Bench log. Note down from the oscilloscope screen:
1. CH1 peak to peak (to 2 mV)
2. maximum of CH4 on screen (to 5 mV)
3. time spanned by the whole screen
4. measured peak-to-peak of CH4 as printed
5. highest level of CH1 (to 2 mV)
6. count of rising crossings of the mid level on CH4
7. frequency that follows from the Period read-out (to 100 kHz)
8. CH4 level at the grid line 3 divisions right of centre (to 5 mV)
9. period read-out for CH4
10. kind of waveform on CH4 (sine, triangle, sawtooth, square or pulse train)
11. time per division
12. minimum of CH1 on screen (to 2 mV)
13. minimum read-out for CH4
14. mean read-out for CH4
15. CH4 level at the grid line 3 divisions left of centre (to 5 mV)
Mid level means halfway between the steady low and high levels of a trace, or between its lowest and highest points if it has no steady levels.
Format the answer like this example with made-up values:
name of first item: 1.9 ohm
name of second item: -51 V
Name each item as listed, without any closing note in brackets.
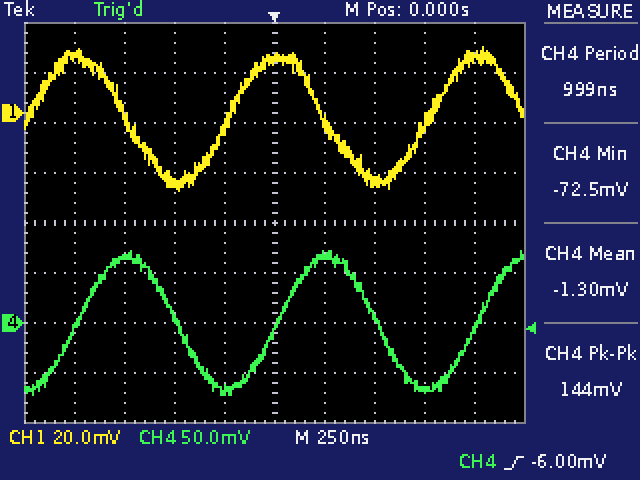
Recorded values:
CH1 peak to peak: 58 mV
maximum of CH4 on screen: 70 mV
time spanned by the whole screen: 2.5 µs
measured peak-to-peak of CH4 as printed: 144 mV
highest level of CH1: 26 mV
count of rising crossings of the mid level on CH4: 3
frequency that follows from the Period read-out: 1.0 MHz
CH4 level at the grid line 3 divisions right of centre: -65 mV
period read-out for CH4: 999 ns
kind of waveform on CH4: sine
time per division: 250 ns
minimum of CH1 on screen: -32 mV
minimum read-out for CH4: -72.5 mV
mean read-out for CH4: -1.30 mV
CH4 level at the grid line 3 divisions left of centre: 65 mV
